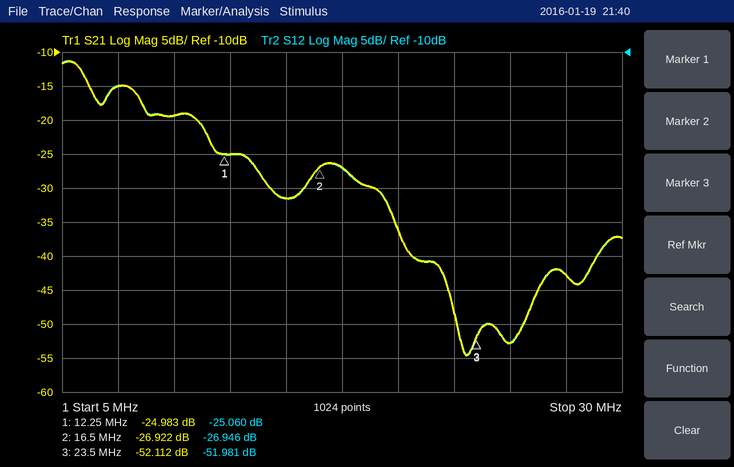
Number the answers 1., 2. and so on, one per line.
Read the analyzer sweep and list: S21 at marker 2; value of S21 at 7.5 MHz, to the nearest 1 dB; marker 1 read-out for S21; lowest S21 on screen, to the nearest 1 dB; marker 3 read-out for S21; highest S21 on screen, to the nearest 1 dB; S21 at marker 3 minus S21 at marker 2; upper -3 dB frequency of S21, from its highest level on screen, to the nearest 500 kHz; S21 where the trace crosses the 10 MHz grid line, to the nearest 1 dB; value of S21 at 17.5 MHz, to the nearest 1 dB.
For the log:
1. -26.922 dB
2. -15 dB
3. -24.983 dB
4. -55 dB
5. -52.112 dB
6. -11 dB
7. -25.190 dB
8. 6.0 MHz
9. -19 dB
10. -27 dB
